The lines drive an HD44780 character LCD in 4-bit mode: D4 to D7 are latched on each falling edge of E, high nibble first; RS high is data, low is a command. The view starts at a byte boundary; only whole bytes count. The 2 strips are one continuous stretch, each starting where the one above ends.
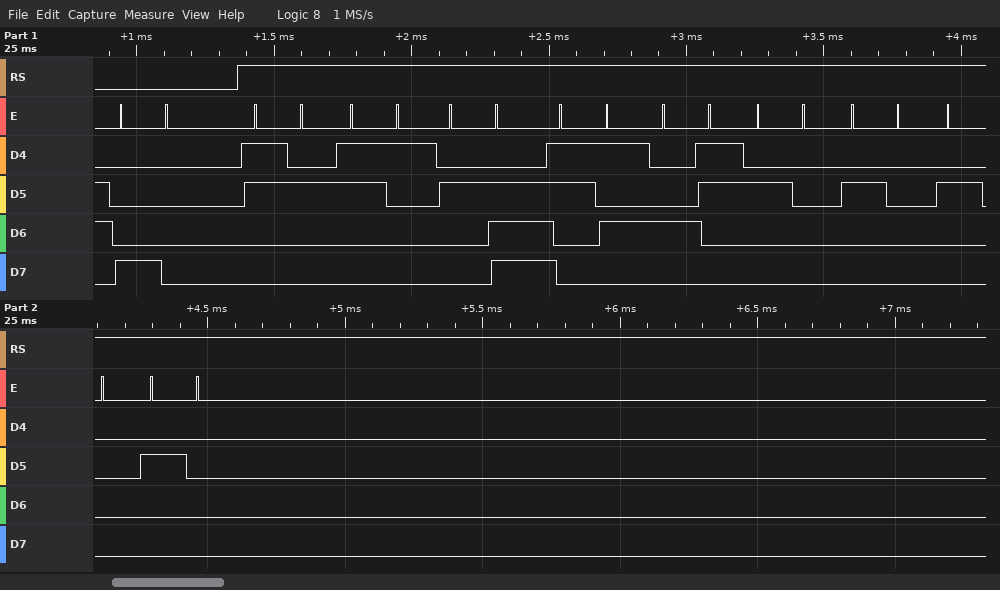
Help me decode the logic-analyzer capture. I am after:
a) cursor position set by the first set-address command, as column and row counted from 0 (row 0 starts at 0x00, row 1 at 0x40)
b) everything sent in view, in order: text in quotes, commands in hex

column 0, row 0
0x80 "21.5C    "
